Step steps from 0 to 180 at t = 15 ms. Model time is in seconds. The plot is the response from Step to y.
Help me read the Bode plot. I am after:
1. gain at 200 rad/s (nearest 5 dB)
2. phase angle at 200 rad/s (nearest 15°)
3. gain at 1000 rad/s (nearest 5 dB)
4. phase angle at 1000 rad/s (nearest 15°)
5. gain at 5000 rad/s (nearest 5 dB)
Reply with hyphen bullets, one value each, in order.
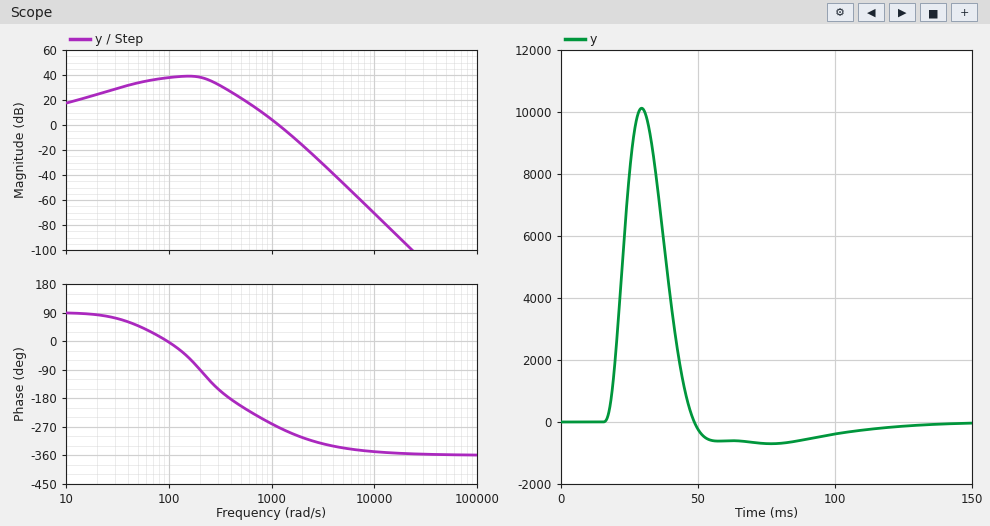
- 40 dB
- -90°
- 5 dB
- -255°
- -45 dB
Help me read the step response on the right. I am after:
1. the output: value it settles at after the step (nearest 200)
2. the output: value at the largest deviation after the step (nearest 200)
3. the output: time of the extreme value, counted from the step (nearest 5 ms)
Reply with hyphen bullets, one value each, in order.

- 0
- 10200
- 15 ms
